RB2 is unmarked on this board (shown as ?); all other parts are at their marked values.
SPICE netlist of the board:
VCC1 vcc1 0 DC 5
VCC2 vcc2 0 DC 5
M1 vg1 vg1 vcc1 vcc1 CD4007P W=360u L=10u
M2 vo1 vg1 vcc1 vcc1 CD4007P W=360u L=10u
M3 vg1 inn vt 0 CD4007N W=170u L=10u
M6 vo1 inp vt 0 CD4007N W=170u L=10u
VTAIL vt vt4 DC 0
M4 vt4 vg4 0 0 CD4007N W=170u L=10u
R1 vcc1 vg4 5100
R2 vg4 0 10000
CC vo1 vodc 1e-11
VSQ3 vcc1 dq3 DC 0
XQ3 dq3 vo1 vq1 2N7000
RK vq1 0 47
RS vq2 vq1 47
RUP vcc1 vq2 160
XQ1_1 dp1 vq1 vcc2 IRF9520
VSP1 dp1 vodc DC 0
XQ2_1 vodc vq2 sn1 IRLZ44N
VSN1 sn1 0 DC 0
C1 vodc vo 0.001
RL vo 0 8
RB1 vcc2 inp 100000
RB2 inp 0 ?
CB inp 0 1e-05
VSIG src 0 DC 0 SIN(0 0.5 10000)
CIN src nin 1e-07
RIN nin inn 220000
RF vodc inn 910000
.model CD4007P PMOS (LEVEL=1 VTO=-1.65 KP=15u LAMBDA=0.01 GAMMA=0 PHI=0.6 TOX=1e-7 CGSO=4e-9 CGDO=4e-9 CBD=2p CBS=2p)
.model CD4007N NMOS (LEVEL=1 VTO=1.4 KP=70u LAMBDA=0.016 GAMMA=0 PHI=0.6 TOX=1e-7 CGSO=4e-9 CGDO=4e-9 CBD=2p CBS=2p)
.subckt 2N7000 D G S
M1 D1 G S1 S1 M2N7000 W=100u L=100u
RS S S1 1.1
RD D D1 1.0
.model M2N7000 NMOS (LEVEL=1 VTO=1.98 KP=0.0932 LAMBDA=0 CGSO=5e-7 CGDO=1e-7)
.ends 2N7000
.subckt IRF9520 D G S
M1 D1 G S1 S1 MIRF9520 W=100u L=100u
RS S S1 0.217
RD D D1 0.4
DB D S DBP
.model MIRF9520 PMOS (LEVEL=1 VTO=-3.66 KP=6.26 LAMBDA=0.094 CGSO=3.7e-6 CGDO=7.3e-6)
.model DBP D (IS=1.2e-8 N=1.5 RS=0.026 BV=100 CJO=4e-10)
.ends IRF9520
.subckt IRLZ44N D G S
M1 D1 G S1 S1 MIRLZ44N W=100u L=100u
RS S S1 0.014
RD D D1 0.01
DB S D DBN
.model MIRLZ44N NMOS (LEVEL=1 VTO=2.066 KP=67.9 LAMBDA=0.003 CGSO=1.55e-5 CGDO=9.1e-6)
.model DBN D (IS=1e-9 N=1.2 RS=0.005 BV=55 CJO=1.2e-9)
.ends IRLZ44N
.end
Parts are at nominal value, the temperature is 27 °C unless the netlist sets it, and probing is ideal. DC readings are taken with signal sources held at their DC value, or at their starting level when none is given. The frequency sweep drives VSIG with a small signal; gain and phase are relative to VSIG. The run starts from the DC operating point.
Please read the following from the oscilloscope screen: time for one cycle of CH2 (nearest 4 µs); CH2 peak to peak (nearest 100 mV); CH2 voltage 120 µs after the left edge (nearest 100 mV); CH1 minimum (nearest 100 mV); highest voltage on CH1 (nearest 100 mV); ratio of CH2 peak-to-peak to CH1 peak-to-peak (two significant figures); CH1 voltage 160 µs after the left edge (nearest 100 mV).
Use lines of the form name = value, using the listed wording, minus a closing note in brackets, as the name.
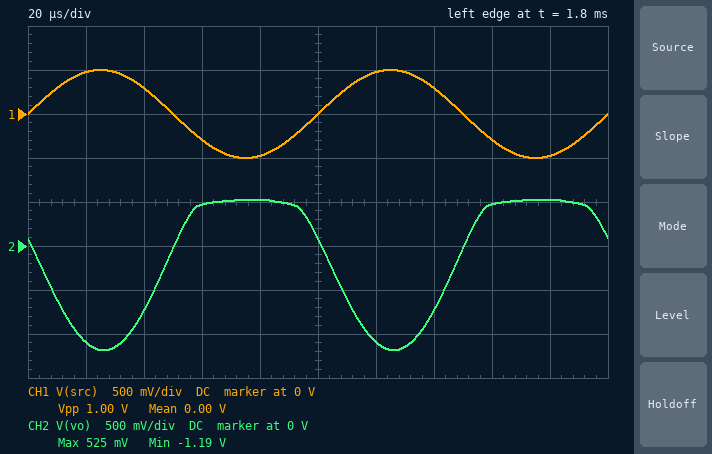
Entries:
time for one cycle of CH2 = 100 µs
CH2 peak to peak = 1.7 V
CH2 voltage 120 µs after the left edge = -1.1 V
CH1 minimum = -500 mV
highest voltage on CH1 = 500 mV
ratio of CH2 peak-to-peak to CH1 peak-to-peak = 1.7
CH1 voltage 160 µs after the left edge = -300 mV
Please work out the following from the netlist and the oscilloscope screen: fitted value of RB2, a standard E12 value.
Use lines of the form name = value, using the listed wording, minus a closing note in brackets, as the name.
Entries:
fitted value of RB2, a standard E12 value = 270 kΩ
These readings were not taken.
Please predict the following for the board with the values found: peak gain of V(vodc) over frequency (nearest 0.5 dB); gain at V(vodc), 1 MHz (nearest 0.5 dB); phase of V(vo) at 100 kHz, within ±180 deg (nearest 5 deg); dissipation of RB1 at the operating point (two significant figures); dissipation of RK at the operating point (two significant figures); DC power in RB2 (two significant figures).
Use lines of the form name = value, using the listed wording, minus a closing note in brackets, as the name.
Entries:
peak gain of V(vodc) over frequency = 10.0 dB
gain at V(vodc), 1 MHz = -14.5 dB
phase of V(vo) at 100 kHz, within ±180 deg = 150 deg
dissipation of RB1 at the operating point = 18 µW
dissipation of RK at the operating point = 33 mW
DC power in RB2 = 49 µW
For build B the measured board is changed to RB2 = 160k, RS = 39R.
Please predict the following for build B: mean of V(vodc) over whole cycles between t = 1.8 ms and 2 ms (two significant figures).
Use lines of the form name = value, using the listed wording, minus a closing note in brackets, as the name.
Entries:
mean of V(vodc) over whole cycles between t = 1.8 ms and 2 ms = 3.1 V
